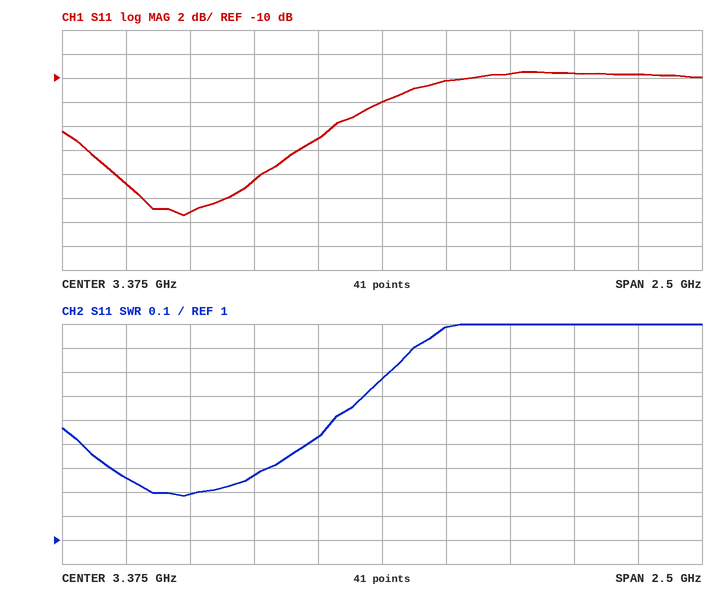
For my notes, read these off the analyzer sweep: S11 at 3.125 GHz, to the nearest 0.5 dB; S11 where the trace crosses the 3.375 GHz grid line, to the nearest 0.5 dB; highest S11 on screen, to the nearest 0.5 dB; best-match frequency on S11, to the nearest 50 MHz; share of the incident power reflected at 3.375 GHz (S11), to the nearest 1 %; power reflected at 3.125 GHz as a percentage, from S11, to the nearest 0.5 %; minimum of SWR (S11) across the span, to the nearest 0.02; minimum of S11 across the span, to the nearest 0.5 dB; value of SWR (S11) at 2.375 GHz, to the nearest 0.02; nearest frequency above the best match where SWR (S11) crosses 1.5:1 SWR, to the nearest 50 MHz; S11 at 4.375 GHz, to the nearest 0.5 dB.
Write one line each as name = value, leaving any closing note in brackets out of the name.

S11 at 3.125 GHz, to the nearest 0.5 dB = -15.0 dB
S11 where the trace crosses the 3.375 GHz grid line, to the nearest 0.5 dB = -12.0 dB
highest S11 on screen, to the nearest 0.5 dB = -9.5 dB
best-match frequency on S11, to the nearest 50 MHz = 2.60 GHz
share of the incident power reflected at 3.375 GHz (S11), to the nearest 1 % = 6 %
power reflected at 3.125 GHz as a percentage, from S11, to the nearest 0.5 % = 3.0 %
minimum of SWR (S11) across the span, to the nearest 0.02 = 1.18
minimum of S11 across the span, to the nearest 0.5 dB = -21.5 dB
value of SWR (S11) at 2.375 GHz, to the nearest 0.02 = 1.26
nearest frequency above the best match where SWR (S11) crosses 1.5:1 SWR, to the nearest 50 MHz = 3.20 GHz
S11 at 4.375 GHz, to the nearest 0.5 dB = -9.5 dB
